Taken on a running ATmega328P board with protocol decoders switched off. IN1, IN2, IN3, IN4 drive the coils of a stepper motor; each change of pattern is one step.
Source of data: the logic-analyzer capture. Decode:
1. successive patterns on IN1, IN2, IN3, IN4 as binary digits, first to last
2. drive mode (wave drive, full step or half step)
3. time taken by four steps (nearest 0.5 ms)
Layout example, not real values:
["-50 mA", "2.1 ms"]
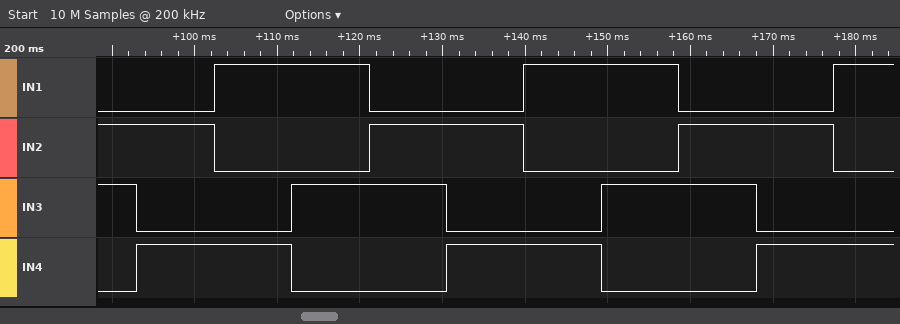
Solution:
["0110 0101 1001 1010 0110 0101 1001 1010 0110 0101 1001", "full step", "37.5 ms"]
